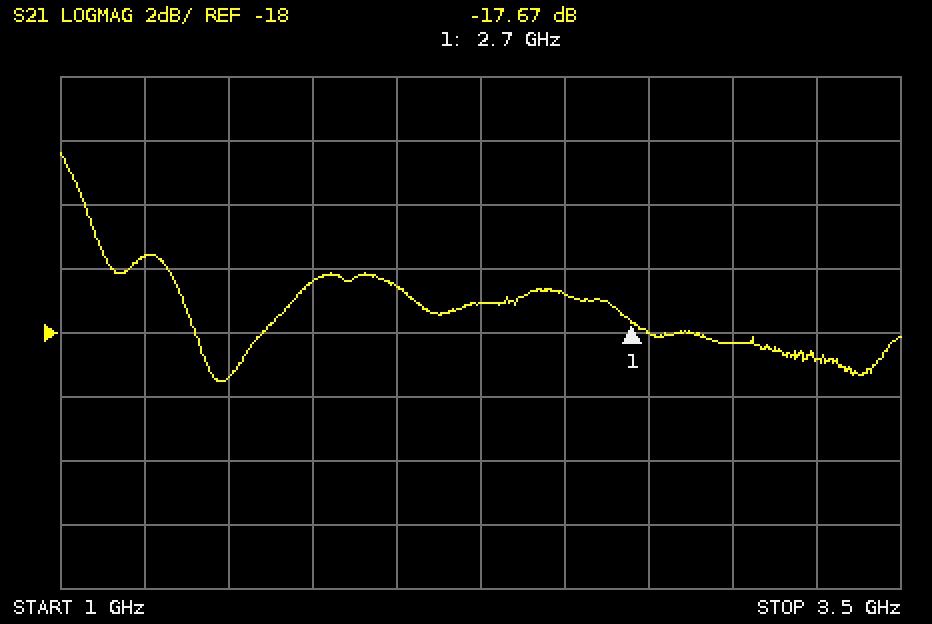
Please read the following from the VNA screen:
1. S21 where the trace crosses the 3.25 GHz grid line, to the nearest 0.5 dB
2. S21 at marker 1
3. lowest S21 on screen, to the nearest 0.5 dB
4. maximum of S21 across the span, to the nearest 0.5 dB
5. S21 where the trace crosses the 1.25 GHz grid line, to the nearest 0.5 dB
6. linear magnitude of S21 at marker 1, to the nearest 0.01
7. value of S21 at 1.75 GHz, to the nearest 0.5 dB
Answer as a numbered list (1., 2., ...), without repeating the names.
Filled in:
1. -19.0 dB
2. -17.67 dB
3. -19.5 dB
4. -12.5 dB
5. -15.5 dB
6. 0.13
7. -16.5 dB
